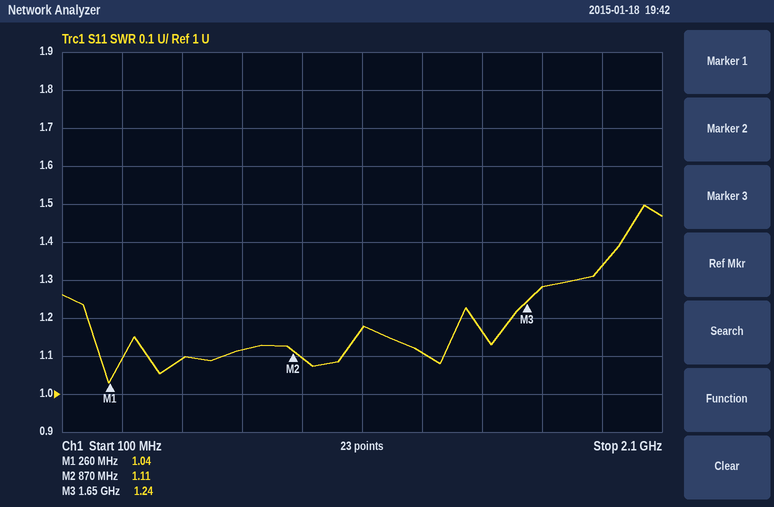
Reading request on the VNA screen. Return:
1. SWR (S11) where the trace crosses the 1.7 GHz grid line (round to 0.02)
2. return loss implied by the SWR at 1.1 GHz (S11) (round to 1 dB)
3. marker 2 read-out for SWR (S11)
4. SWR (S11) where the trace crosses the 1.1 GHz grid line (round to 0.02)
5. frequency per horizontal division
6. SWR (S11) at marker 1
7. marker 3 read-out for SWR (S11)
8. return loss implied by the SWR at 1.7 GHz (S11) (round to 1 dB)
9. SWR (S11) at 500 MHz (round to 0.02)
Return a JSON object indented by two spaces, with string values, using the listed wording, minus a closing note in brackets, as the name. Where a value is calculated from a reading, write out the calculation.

{
  "SWR (S11) where the trace crosses the 1.7 GHz grid line": "1.28",
  "return loss implied by the SWR at 1.1 GHz (S11)": "−20 log10((1.18 − 1)/(1.18 + 1)) ≈ 22 dB",
  "marker 2 read-out for SWR": "1.11",
  "SWR (S11) where the trace crosses the 1.1 GHz grid line": "1.18",
  "frequency per horizontal division": "200 MHz",
  "SWR (S11) at marker 1": "1.04",
  "marker 3 read-out for SWR": "1.24",
  "return loss implied by the SWR at 1.7 GHz (S11)": "−20 log10((1.28 − 1)/(1.28 + 1)) ≈ 18 dB",
  "SWR (S11) at 500 MHz": "1.10"
}
